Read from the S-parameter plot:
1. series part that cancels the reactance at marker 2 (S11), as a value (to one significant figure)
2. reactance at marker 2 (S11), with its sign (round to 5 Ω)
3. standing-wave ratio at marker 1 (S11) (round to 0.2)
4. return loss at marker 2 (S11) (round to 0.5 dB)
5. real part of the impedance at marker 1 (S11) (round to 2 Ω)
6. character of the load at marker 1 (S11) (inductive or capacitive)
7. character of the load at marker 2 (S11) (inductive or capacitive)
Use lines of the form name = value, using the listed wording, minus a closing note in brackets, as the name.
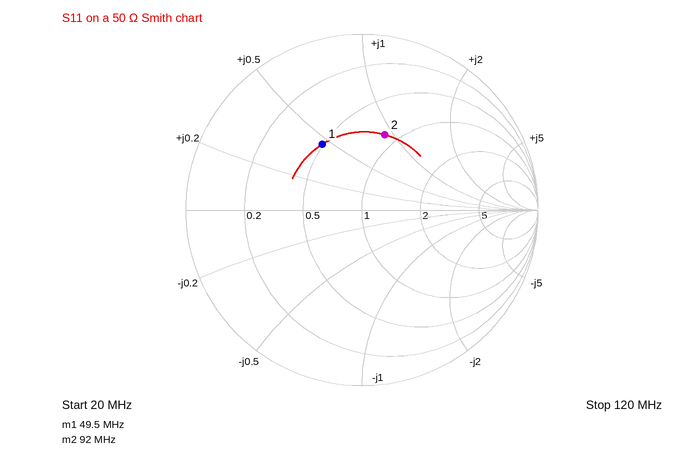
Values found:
series part that cancels the reactance at marker 2 (S11), as a value = 40 pF
reactance at marker 2 (S11), with its sign = +45 Ω
standing-wave ratio at marker 1 (S11) = 2.6
return loss at marker 2 (S11) = 7.0 dB
real part of the impedance at marker 1 (S11) = 24 Ω
character of the load at marker 1 (S11) = inductive
character of the load at marker 2 (S11) = inductive
